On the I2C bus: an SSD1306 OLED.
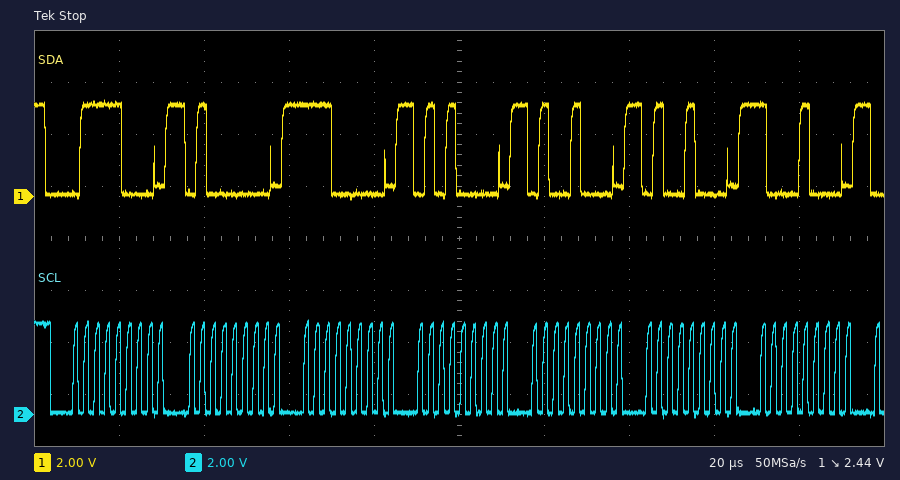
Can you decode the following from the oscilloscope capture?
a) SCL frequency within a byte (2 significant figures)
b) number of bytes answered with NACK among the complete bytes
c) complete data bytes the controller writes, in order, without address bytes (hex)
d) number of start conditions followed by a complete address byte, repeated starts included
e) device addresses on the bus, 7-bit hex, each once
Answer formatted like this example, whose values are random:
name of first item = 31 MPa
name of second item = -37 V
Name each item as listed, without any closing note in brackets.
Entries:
SCL frequency within a byte = 400 kHz
number of bytes answered with NACK among the complete bytes = 0
complete data bytes the controller writes, in order, without address bytes = 40 E0 50 48 48 88
number of start conditions followed by a complete address byte, repeated starts included = 1
device addresses on the bus, 7-bit hex, each once = 0x3C
